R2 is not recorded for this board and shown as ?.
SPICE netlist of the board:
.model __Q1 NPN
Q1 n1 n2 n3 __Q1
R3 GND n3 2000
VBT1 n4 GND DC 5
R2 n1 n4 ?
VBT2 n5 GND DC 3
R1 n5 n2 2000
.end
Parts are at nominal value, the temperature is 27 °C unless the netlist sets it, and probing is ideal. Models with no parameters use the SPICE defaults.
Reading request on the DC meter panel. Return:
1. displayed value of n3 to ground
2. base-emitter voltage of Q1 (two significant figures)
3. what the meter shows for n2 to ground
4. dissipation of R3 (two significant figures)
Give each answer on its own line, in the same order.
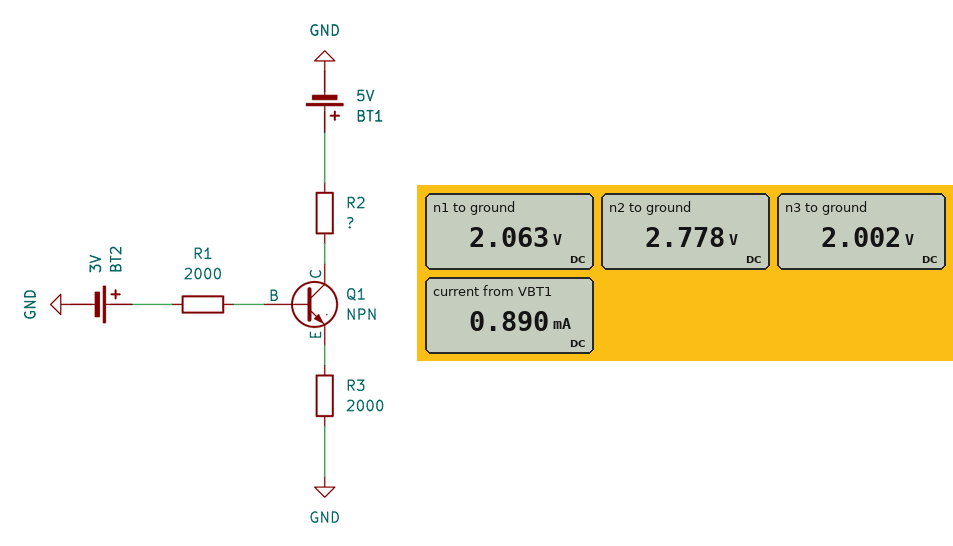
2.002 V
780 mV
2.778 V
2.0 mW
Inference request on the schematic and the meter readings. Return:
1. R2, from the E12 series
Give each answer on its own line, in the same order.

3.3 kΩ
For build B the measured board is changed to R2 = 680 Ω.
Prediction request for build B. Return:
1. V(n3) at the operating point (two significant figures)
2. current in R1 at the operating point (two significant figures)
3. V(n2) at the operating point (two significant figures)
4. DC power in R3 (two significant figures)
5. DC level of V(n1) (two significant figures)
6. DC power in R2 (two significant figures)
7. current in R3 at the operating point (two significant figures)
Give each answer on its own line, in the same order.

2.2 V
11 µA
3.0 V
2.4 mW
4.3 V
810 µW
1.1 mA
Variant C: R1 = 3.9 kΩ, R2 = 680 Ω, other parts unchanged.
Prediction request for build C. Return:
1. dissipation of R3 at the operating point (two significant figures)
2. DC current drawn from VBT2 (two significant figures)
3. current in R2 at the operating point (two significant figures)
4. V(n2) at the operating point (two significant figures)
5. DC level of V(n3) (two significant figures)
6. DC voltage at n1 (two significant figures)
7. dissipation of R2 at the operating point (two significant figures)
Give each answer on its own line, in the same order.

2.4 mW
11 µA
1.1 mA
3.0 V
2.2 V
4.3 V
790 µW
